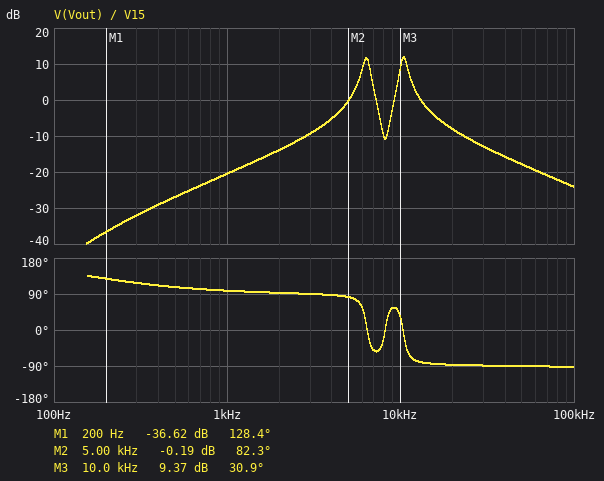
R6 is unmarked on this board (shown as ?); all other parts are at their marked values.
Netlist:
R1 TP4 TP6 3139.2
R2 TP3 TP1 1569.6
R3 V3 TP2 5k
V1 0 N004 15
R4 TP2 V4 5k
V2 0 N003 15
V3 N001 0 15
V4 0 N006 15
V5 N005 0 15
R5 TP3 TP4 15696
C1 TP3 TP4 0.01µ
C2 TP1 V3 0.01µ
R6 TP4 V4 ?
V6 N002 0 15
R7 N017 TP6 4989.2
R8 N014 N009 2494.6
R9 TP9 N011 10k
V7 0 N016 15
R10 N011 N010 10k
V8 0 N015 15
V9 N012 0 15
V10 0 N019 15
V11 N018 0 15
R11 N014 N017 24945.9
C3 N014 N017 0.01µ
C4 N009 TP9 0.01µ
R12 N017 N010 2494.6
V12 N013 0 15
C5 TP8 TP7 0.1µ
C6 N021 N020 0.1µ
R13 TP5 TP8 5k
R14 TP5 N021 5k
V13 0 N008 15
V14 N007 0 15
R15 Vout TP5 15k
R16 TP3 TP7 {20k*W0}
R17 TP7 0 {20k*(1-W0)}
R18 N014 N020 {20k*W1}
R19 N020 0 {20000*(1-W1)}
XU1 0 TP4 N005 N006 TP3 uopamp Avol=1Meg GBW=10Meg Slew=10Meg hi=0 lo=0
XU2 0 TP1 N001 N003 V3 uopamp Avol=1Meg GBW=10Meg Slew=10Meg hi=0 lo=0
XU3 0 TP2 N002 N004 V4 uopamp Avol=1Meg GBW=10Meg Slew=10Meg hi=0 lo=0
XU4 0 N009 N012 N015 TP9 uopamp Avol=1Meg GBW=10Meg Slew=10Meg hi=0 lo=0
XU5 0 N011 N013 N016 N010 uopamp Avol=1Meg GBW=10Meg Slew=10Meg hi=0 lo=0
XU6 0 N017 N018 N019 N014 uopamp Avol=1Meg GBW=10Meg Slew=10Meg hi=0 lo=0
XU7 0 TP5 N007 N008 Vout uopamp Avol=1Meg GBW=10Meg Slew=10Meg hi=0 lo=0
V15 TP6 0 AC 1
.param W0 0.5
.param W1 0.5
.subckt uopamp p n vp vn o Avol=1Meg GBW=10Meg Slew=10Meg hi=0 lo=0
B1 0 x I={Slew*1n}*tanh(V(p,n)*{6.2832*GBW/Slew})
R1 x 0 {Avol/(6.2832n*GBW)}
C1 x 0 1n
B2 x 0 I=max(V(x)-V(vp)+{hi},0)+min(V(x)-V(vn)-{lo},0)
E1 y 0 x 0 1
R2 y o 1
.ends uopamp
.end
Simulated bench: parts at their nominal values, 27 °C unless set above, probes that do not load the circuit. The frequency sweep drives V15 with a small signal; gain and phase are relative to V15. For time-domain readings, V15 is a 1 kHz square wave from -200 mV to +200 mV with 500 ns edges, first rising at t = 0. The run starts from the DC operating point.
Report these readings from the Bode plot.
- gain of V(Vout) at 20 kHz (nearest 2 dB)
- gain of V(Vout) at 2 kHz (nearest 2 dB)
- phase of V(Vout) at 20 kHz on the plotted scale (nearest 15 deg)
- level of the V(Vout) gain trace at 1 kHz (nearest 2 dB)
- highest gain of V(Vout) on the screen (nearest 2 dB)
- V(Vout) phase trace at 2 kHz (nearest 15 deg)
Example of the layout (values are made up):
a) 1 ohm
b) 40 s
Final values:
a) -8 dB
b) -14 dB
c) -90 deg
d) -20 dB
e) 12 dB
f) 90 deg
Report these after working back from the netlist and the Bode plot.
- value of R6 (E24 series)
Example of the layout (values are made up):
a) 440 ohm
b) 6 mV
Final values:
a) 1.5 kΩ
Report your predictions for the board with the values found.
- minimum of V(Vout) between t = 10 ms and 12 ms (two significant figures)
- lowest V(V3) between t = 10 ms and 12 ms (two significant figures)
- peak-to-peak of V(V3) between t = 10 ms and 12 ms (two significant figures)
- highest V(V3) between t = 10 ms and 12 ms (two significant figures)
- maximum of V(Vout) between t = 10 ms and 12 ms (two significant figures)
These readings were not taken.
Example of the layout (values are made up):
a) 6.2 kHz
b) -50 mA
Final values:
a) -210 mV
b) -240 mV
c) 480 mV
d) 240 mV
e) 210 mV
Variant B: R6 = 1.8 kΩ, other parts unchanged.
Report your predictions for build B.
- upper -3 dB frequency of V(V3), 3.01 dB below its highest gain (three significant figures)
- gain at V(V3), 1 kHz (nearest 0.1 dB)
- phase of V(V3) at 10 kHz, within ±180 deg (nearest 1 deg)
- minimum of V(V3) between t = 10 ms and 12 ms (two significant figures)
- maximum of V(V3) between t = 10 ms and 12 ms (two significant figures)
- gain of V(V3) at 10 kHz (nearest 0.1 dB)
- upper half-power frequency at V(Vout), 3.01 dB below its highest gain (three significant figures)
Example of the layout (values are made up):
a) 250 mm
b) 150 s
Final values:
a) 9.91 kHz
b) -4.7 dB
c) -137 deg
d) -320 mV
e) 320 mV
f) 11.0 dB
g) 10.1 kHz
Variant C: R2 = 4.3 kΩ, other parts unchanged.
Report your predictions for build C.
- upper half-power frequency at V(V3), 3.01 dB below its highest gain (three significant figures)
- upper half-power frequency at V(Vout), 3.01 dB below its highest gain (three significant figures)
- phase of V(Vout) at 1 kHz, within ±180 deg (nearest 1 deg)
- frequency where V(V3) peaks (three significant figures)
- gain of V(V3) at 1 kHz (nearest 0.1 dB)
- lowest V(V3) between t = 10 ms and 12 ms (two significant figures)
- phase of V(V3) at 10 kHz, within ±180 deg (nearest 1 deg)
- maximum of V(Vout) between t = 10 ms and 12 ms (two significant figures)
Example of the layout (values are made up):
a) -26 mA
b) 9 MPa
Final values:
a) 6.70 kHz
b) 6.74 kHz
c) 98 deg
d) 6.22 kHz
e) -6.2 dB
f) -220 mV
g) -171 deg
h) 290 mV
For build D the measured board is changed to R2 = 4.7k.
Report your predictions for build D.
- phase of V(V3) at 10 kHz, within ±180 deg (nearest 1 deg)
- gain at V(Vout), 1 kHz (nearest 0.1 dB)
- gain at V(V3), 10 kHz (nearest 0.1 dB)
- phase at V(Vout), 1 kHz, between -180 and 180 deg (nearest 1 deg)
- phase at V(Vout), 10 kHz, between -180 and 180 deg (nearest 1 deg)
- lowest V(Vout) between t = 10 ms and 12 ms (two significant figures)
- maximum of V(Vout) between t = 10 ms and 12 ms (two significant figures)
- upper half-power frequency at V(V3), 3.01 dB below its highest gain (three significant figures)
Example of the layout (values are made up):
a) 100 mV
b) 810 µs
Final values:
a) -171 deg
b) -15.5 dB
c) -11.6 dB
d) 98 deg
e) -82 deg
f) -290 mV
g) 290 mV
h) 6.43 kHz
